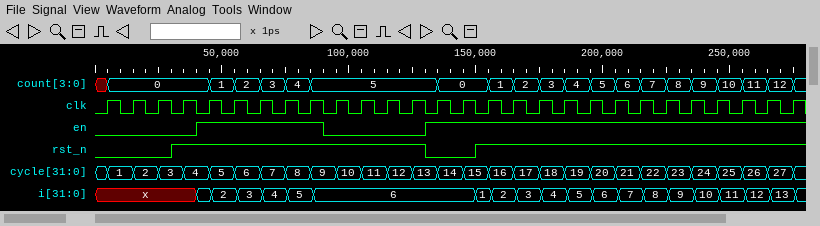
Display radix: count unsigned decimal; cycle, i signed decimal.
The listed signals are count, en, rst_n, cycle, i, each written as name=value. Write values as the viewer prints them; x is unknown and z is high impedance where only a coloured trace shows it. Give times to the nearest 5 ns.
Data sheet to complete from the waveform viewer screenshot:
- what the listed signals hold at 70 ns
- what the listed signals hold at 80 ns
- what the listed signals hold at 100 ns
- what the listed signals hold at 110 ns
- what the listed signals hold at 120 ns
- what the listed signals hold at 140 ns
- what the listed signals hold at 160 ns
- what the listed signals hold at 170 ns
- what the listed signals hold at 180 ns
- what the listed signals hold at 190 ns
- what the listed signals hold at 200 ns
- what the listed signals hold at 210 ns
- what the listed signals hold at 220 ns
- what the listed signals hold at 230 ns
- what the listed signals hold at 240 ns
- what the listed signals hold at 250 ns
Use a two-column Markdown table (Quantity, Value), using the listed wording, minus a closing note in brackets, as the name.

| Quantity | Value |
|---|---|
| what the listed signals hold at 70 ns | count=3, en=1, rst_n=1, cycle=7, i=4 |
| what the listed signals hold at 80 ns | count=4, en=1, rst_n=1, cycle=8, i=5 |
| what the listed signals hold at 100 ns | count=5, en=0, rst_n=1, cycle=10, i=6 |
| what the listed signals hold at 110 ns | count=5, en=0, rst_n=1, cycle=11, i=6 |
| what the listed signals hold at 120 ns | count=5, en=0, rst_n=1, cycle=12, i=6 |
| what the listed signals hold at 140 ns | count=0, en=1, rst_n=0, cycle=14, i=6 |
| what the listed signals hold at 160 ns | count=1, en=1, rst_n=1, cycle=16, i=2 |
| what the listed signals hold at 170 ns | count=2, en=1, rst_n=1, cycle=17, i=3 |
| what the listed signals hold at 180 ns | count=3, en=1, rst_n=1, cycle=18, i=4 |
| what the listed signals hold at 190 ns | count=4, en=1, rst_n=1, cycle=19, i=5 |
| what the listed signals hold at 200 ns | count=5, en=1, rst_n=1, cycle=20, i=6 |
| what the listed signals hold at 210 ns | count=6, en=1, rst_n=1, cycle=21, i=7 |
| what the listed signals hold at 220 ns | count=7, en=1, rst_n=1, cycle=22, i=8 |
| what the listed signals hold at 230 ns | count=8, en=1, rst_n=1, cycle=23, i=9 |
| what the listed signals hold at 240 ns | count=9, en=1, rst_n=1, cycle=24, i=10 |
| what the listed signals hold at 250 ns | count=10, en=1, rst_n=1, cycle=25, i=11 |
